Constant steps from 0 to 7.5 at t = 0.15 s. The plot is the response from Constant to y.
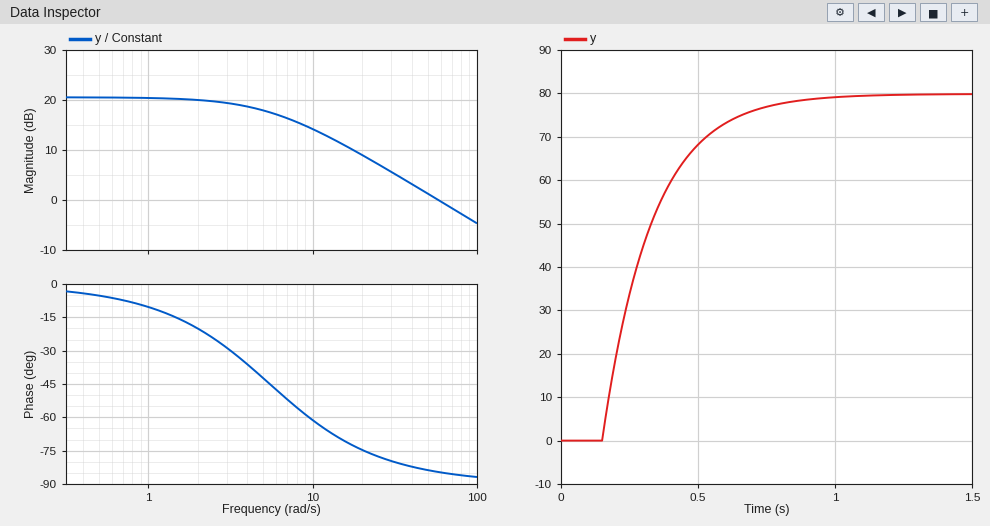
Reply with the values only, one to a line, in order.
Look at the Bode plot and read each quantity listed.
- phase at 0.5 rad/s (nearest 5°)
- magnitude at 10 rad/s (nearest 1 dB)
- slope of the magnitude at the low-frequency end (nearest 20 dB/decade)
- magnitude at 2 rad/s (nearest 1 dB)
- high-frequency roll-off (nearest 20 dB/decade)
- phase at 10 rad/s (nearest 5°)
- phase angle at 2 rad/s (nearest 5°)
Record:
-5°
14 dB
0 dB/decade
20 dB
-20 dB/decade
-60°
-20°
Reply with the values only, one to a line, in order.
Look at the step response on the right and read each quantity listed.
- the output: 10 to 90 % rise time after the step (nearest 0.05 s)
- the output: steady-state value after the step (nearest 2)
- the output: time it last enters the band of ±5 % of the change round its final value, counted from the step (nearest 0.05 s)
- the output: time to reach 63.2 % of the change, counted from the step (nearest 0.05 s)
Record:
0.40 s
80
0.55 s
0.20 s
